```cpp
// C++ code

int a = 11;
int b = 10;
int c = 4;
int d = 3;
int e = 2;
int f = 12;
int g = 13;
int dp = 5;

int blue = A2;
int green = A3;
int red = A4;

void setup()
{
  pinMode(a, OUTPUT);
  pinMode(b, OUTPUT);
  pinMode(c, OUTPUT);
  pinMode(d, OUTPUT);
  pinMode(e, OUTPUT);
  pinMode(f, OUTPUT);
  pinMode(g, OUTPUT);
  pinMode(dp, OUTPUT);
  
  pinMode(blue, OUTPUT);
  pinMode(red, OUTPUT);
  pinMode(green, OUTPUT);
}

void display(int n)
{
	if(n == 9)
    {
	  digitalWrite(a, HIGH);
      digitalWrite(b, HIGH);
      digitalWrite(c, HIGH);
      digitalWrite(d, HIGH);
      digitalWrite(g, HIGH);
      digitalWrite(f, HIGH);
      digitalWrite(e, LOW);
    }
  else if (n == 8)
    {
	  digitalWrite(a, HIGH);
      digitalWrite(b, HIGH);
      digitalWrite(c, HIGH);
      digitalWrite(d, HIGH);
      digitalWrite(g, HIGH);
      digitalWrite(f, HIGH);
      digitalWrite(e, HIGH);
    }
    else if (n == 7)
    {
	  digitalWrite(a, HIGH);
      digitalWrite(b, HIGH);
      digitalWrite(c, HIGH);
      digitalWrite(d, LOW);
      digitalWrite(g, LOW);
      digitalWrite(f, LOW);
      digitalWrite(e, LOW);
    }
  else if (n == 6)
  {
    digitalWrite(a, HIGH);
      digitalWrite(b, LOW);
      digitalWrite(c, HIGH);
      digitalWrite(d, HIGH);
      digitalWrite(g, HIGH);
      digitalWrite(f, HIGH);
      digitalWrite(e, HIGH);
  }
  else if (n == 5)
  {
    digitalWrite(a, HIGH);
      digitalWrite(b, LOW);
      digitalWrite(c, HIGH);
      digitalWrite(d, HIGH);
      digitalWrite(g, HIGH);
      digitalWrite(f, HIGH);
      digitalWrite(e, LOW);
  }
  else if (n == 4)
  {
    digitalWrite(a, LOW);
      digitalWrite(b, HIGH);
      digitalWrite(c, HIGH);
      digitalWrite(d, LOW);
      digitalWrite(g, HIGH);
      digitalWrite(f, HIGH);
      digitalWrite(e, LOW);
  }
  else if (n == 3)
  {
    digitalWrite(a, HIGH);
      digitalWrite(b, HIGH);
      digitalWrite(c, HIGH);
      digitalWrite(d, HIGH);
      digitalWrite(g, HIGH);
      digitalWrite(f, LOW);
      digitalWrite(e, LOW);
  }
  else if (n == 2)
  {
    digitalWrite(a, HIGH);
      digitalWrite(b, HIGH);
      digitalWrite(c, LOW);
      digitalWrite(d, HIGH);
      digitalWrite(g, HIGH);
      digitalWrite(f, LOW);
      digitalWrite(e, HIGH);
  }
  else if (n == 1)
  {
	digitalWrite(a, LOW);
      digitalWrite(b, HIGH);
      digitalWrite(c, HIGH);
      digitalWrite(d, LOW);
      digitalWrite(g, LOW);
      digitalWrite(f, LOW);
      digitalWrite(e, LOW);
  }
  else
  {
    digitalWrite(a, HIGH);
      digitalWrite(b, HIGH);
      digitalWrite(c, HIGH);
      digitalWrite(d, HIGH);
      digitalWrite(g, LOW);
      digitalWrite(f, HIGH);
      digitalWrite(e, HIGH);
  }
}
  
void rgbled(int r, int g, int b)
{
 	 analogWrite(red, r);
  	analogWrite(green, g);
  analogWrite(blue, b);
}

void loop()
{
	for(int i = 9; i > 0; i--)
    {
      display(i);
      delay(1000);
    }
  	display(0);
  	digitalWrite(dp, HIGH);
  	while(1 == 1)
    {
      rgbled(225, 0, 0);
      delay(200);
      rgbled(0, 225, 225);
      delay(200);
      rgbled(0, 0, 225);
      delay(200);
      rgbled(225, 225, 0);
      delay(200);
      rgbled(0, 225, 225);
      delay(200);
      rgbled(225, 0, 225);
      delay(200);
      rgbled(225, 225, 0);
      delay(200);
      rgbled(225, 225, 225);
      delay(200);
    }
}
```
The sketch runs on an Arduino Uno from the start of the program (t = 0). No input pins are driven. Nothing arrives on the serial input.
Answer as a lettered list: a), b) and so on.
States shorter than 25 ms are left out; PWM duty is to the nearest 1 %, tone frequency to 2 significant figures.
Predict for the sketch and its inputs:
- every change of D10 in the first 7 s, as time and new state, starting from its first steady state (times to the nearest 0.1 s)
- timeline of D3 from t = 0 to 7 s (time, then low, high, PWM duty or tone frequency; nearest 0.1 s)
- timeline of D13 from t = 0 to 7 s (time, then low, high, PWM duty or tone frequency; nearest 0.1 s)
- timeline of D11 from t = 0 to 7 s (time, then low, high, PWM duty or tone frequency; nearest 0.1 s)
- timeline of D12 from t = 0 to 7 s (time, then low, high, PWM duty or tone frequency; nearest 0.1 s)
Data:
a) 0 s high; 3 s low; 5 s high
b) 0 s high; 2 s low; 3 s high; 5 s low; 6 s high
c) 0 s high; 2 s low; 3 s high
d) 0 s high; 5 s low; 6 s high
e) 0 s high; 2 s low; 3 s high; 6 s low
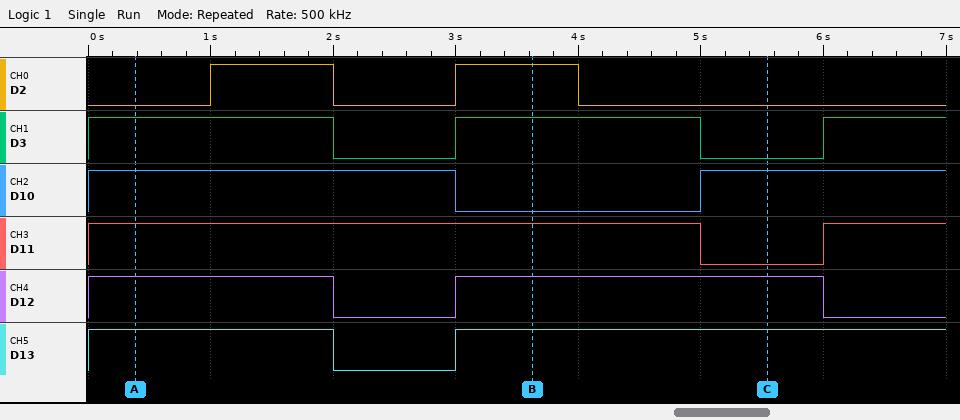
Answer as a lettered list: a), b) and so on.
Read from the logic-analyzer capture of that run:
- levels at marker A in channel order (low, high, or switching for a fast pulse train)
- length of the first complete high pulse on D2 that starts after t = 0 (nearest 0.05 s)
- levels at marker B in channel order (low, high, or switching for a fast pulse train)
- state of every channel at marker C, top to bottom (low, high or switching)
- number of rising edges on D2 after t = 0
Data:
a) D2 low, D3 high, D10 high, D11 high, D12 high, D13 high
b) 1.00 s
c) D2 high, D3 high, D10 low, D11 high, D12 high, D13 high
d) D2 low, D3 low, D10 high, D11 low, D12 high, D13 high
e) 2
